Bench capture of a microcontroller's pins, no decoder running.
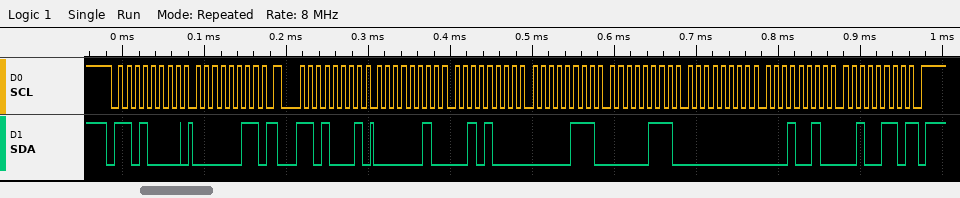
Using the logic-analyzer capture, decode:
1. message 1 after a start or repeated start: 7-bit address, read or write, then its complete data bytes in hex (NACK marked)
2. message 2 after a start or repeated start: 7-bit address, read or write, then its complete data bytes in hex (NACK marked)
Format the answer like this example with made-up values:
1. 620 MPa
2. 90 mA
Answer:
1. 0x68 write: 03
2. 0x68 read: 02 28 07 07 00 12 26 NACK
